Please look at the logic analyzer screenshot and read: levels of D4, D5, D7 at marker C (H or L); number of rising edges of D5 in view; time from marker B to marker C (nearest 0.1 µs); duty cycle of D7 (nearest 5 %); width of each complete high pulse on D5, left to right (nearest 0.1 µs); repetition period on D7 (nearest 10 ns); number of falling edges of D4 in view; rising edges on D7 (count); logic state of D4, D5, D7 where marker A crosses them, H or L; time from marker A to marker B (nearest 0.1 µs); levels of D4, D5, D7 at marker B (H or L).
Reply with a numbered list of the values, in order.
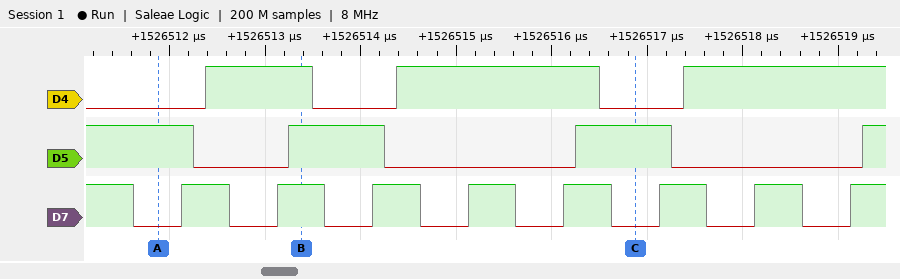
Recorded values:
1. D4=L, D5=H, D7=L
2. 3
3. 3.5 µs
4. 50 %
5. 1 µs, 1 µs
6. 1000 ns
7. 2
8. 8
9. D4=L, D5=H, D7=L
10. 1.5 µs
11. D4=H, D5=H, D7=H
